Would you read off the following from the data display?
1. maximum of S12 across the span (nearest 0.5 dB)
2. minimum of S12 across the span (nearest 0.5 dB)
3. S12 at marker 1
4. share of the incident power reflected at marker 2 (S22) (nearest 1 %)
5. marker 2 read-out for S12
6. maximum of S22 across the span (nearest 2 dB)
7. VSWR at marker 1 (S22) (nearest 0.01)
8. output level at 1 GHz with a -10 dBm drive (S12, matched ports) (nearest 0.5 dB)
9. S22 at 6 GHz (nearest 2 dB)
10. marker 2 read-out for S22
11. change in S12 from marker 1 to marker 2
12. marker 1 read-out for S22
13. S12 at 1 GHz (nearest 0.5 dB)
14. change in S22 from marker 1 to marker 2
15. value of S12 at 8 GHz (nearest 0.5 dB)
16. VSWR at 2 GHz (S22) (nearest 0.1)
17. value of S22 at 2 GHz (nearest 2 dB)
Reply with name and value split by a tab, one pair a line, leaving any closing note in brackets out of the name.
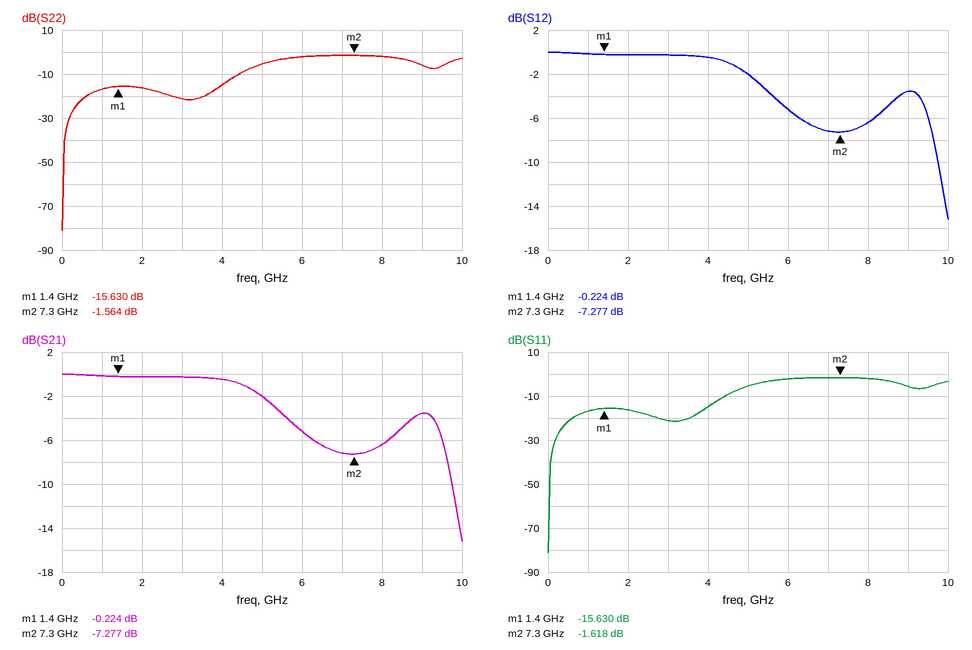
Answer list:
maximum of S12 across the span	0.0 dB
minimum of S12 across the span	-15.0 dB
S12 at marker 1	-0.224 dB
share of the incident power reflected at marker 2 (S22)	70 %
marker 2 read-out for S12	-7.277 dB
maximum of S22 across the span	-2 dB
VSWR at marker 1 (S22)	1.40
output level at 1 GHz with a -10 dBm drive (S12, matched ports)	-10.0 dBm
S22 at 6 GHz	-2 dB
marker 2 read-out for S22	-1.564 dB
change in S12 from marker 1 to marker 2	-7.053 dB
marker 1 read-out for S22	-15.630 dB
S12 at 1 GHz	0.0 dB
change in S22 from marker 1 to marker 2	14.066 dB
value of S12 at 8 GHz	-6.5 dB
VSWR at 2 GHz (S22)	1.4
value of S22 at 2 GHz	-16 dB
